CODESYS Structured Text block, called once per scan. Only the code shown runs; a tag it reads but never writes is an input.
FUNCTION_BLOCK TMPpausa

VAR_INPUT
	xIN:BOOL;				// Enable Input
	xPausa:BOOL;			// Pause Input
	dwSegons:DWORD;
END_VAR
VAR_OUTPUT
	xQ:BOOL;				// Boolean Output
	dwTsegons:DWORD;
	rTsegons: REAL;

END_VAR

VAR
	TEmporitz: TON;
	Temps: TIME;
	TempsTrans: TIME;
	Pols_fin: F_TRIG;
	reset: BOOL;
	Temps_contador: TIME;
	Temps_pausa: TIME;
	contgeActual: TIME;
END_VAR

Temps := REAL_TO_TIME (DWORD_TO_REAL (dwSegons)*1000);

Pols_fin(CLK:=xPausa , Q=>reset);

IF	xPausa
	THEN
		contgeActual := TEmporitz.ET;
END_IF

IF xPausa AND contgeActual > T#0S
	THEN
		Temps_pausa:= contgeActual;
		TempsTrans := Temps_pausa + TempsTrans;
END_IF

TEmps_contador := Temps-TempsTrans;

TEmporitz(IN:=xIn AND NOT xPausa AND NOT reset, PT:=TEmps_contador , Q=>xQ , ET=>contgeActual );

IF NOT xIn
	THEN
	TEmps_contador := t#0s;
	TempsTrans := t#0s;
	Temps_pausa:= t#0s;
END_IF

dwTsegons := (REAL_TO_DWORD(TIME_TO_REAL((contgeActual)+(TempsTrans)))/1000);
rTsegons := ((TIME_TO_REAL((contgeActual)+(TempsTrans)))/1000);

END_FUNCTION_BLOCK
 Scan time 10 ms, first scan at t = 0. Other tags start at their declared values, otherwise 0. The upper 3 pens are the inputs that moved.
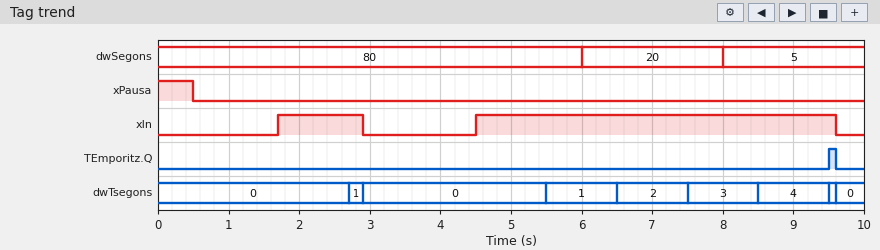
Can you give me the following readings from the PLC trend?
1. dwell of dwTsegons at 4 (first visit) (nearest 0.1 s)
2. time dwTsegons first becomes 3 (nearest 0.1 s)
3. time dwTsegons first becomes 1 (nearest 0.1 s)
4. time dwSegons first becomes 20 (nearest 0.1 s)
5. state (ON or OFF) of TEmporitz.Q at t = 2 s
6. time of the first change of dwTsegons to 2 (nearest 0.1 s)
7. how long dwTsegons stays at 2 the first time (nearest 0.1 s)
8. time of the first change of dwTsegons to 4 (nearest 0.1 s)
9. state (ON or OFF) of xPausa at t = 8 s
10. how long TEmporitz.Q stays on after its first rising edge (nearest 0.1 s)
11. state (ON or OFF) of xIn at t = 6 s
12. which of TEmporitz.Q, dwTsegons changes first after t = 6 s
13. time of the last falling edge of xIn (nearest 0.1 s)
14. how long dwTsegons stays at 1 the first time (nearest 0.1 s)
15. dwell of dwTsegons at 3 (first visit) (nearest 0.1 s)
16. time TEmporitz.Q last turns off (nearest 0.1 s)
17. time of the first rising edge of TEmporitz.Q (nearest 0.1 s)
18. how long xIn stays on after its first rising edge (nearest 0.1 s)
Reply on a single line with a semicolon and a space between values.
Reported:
1.0 s; 7.5 s; 2.7 s; 6.0 s; OFF; 6.5 s; 1.0 s; 8.5 s; OFF; 0.1 s; ON; dwTsegons; 9.6 s; 0.2 s; 1.0 s; 9.6 s; 9.5 s; 1.2 s
